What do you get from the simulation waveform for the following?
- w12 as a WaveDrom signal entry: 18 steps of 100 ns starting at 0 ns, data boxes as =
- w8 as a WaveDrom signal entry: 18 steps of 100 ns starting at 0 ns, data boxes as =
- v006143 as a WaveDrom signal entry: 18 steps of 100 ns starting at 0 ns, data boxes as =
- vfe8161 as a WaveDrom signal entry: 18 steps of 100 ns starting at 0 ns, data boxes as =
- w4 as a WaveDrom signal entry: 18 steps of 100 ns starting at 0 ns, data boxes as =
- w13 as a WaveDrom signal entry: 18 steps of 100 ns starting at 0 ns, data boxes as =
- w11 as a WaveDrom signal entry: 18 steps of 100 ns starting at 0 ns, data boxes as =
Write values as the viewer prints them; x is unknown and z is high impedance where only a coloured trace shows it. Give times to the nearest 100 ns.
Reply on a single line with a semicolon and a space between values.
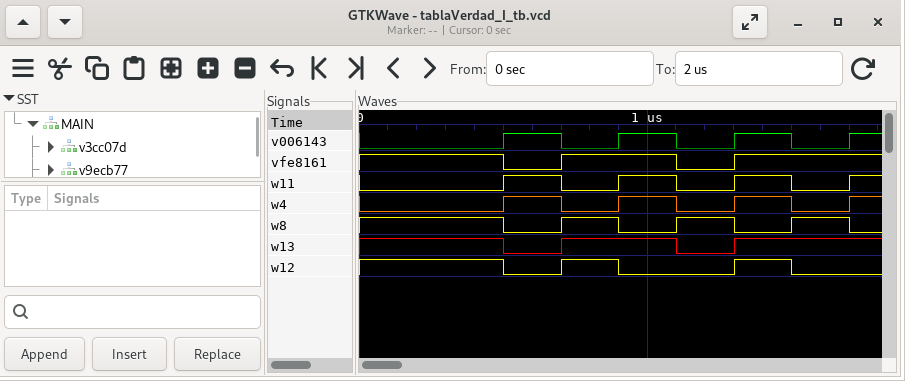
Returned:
{name: 'w12', wave: '1....0.1.0...1.0..'}; {name: 'w8', wave: '1....0.1.0.1.0.1.0'}; {name: 'v006143', wave: '0....1.0.1.0.1.0.1'}; {name: 'vfe8161', wave: '1....0.1...0.1....'}; {name: 'w4', wave: '0....1.0.1.0.1.0.1'}; {name: 'w13', wave: '1....0.1...0.1....'}; {name: 'w11', wave: '0....1.0.1.0.1.0.1'}
